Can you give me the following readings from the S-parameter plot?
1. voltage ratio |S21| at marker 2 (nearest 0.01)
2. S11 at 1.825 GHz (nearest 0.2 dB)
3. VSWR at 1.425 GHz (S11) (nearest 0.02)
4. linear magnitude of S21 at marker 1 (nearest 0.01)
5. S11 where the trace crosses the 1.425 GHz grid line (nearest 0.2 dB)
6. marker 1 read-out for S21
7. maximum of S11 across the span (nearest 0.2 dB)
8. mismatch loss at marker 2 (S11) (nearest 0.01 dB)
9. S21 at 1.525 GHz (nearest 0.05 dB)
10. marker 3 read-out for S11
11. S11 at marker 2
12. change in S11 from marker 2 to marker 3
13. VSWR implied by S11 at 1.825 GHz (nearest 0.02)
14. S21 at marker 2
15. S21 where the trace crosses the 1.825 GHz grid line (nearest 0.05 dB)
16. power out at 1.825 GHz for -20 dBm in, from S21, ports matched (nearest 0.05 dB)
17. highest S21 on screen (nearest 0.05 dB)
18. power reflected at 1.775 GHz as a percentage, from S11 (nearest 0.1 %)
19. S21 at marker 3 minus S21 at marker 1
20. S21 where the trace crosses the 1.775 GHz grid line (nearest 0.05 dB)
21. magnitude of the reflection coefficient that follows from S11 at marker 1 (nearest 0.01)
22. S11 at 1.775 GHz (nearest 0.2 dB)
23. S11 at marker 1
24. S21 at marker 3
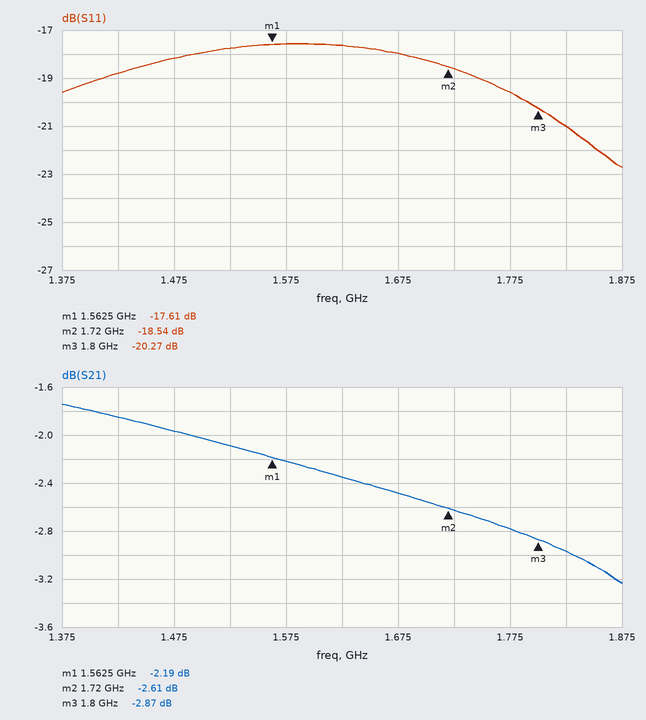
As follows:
0.74
-21.0 dB
1.26
0.78
-18.8 dB
-2.19 dB
-17.6 dB
0.06 dB
-2.10 dB
-20.27 dB
-18.54 dB
-1.73 dB
1.20
-2.61 dB
-2.95 dB
-22.95 dBm
-1.75 dB
1.1 %
-0.68 dB
-2.80 dB
0.13
-19.6 dB
-17.61 dB
-2.87 dB
